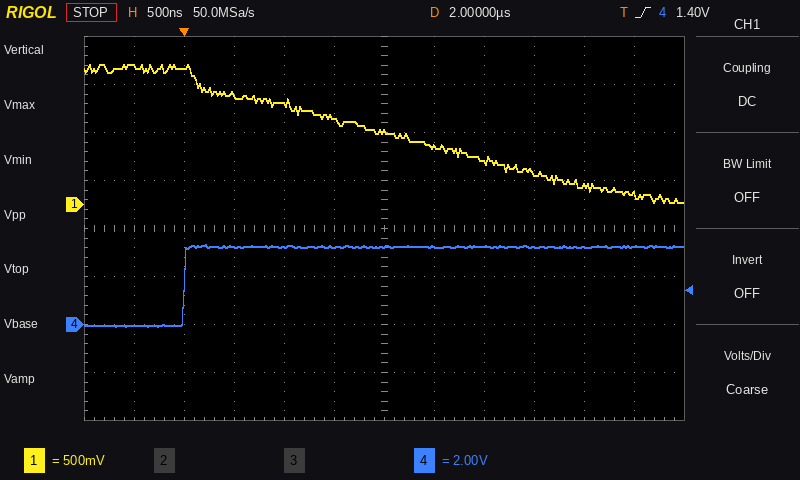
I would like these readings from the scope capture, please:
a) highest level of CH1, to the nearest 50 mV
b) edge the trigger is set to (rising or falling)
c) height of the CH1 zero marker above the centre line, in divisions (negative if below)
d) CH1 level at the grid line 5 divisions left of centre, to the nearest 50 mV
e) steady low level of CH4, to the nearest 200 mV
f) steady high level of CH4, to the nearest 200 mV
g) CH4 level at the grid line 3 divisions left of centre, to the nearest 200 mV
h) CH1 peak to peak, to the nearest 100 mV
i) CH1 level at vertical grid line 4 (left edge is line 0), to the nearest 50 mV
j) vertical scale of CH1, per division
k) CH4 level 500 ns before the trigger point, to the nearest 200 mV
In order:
1.45 V
rising
+0.5 div
1.45 V
0.0 V
3.2 V
3.2 V
1.40 V
1.05 V
500 mV
0.0 V
